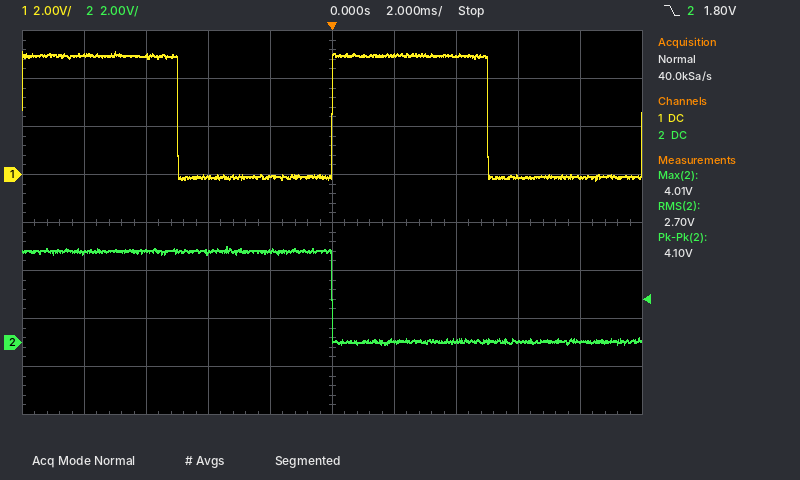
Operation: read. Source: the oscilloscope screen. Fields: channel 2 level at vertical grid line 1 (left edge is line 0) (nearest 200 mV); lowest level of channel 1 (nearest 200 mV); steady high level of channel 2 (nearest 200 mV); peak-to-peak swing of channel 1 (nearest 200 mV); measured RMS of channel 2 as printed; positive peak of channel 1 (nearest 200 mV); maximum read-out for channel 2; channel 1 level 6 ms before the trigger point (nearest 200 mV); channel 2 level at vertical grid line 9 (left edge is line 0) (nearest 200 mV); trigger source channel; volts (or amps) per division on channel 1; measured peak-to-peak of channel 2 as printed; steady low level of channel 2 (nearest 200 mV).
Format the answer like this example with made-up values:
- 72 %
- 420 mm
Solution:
- 3.8 V
- -200 mV
- 3.8 V
- 5.4 V
- 2.70 V
- 5.2 V
- 4.01 V
- 5.0 V
- 0.0 V
- channel 2
- 2 V
- 4.10 V
- 0.0 V
